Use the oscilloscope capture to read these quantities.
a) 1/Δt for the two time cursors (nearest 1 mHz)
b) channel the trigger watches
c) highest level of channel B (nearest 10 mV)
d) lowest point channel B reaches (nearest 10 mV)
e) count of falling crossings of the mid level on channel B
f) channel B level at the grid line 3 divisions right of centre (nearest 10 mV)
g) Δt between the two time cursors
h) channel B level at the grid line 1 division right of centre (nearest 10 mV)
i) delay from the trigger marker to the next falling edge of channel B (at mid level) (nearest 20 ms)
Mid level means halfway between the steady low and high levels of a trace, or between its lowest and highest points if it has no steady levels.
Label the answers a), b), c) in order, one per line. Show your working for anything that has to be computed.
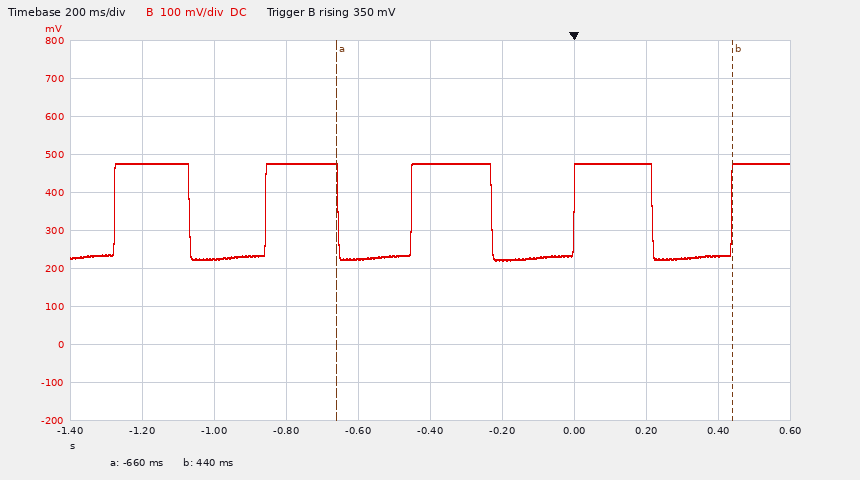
a) 1 / 1.10 s ≈ 909 mHz
b) channel B
c) 480 mV
d) 220 mV
e) 4
f) 480 mV
g) 440 ms − (-660 ms) = 1.10 s
h) 220 mV
i) 220 ms
